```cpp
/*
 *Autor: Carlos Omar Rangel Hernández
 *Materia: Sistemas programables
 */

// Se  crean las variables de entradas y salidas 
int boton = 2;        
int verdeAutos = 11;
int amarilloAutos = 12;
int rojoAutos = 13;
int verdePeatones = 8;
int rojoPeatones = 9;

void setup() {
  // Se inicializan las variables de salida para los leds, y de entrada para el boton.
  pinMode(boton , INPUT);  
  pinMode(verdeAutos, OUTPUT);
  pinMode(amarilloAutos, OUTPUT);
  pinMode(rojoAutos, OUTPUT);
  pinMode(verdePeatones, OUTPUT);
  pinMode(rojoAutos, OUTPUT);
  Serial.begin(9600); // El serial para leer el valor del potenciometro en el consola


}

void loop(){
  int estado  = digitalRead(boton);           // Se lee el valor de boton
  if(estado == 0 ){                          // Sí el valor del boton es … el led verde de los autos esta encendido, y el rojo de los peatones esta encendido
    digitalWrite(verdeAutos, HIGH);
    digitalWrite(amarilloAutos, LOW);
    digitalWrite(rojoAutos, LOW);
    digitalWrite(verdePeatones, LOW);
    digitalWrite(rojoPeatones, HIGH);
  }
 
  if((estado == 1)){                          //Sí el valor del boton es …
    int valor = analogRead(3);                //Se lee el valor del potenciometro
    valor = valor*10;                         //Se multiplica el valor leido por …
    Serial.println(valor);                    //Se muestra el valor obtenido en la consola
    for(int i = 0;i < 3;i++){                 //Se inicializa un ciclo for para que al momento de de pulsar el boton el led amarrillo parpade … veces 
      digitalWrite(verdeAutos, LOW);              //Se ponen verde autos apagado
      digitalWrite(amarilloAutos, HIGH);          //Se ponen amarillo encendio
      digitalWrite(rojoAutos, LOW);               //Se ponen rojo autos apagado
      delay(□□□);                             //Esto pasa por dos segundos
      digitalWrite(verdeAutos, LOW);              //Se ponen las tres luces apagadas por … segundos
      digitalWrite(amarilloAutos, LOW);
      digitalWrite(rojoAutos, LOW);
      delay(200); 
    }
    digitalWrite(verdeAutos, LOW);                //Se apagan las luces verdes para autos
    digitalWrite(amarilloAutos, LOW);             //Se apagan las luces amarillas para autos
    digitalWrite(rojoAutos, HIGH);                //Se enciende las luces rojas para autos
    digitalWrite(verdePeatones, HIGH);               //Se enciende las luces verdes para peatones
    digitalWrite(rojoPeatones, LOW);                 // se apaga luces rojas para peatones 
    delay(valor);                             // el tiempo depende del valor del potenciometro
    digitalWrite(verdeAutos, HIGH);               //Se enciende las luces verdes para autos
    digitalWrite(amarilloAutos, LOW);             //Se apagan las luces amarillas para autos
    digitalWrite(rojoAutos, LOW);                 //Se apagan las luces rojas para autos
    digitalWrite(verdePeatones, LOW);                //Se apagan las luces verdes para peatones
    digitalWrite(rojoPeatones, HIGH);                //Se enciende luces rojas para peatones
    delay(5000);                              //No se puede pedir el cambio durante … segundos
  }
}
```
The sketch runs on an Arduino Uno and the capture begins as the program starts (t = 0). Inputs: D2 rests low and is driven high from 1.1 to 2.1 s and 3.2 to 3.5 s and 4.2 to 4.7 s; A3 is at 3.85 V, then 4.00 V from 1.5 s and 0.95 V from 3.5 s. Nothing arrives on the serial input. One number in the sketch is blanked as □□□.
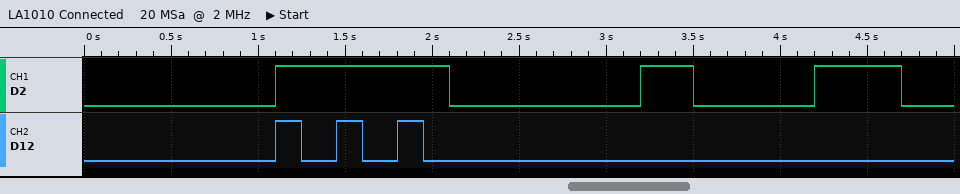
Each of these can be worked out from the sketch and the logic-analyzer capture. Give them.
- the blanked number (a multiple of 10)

150
